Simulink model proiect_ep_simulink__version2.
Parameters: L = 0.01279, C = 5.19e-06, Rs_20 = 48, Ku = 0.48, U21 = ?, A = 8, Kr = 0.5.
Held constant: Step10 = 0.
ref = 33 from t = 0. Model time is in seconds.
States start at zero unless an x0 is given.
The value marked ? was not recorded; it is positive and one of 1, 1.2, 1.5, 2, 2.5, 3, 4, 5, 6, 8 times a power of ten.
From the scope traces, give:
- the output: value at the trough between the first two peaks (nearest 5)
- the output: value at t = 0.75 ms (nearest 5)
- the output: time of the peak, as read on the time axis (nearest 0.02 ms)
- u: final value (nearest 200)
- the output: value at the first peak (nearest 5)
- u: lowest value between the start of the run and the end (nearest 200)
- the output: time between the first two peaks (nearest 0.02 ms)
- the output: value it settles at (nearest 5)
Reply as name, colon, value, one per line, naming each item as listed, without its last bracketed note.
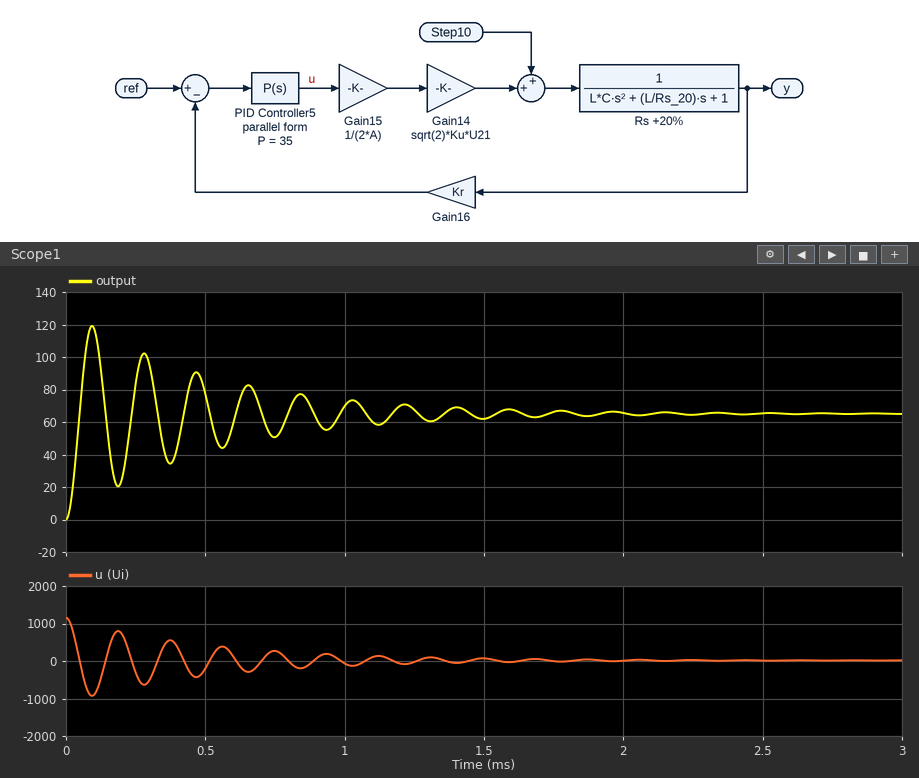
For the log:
the output: value at the trough between the first two peaks: 20
the output: value at t = 0.75 ms: 50
the output: time of the peak, as read on the time axis: 0.10 ms
u: final value: 0
the output: value at the first peak: 120
u: lowest value between the start of the run and the end: -1000
the output: time between the first two peaks: 0.18 ms
the output: value it settles at: 65
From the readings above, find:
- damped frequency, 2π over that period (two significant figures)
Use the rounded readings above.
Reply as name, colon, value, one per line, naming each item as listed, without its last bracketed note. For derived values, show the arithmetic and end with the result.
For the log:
damped frequency, 2π over that period: 2π / 0.18 = 35 rad/ms
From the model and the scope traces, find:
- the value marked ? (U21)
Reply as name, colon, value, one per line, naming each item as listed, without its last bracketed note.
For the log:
the value marked ?: 100
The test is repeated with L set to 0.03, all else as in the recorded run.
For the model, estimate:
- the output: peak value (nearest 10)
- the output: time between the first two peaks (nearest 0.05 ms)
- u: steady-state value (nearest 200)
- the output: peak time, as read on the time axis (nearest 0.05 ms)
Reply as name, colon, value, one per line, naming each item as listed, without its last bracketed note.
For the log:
the output: peak value: 110
the output: time between the first two peaks: 0.30 ms
u: steady-state value: 0
the output: peak time, as read on the time axis: 0.15 ms
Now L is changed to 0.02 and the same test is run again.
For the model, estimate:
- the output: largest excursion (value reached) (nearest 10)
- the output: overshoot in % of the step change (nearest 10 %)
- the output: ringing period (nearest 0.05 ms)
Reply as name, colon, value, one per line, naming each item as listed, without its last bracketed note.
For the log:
the output: largest excursion (value reached): 120
the output: overshoot in % of the step change: 80 %
the output: ringing period: 0.25 ms
